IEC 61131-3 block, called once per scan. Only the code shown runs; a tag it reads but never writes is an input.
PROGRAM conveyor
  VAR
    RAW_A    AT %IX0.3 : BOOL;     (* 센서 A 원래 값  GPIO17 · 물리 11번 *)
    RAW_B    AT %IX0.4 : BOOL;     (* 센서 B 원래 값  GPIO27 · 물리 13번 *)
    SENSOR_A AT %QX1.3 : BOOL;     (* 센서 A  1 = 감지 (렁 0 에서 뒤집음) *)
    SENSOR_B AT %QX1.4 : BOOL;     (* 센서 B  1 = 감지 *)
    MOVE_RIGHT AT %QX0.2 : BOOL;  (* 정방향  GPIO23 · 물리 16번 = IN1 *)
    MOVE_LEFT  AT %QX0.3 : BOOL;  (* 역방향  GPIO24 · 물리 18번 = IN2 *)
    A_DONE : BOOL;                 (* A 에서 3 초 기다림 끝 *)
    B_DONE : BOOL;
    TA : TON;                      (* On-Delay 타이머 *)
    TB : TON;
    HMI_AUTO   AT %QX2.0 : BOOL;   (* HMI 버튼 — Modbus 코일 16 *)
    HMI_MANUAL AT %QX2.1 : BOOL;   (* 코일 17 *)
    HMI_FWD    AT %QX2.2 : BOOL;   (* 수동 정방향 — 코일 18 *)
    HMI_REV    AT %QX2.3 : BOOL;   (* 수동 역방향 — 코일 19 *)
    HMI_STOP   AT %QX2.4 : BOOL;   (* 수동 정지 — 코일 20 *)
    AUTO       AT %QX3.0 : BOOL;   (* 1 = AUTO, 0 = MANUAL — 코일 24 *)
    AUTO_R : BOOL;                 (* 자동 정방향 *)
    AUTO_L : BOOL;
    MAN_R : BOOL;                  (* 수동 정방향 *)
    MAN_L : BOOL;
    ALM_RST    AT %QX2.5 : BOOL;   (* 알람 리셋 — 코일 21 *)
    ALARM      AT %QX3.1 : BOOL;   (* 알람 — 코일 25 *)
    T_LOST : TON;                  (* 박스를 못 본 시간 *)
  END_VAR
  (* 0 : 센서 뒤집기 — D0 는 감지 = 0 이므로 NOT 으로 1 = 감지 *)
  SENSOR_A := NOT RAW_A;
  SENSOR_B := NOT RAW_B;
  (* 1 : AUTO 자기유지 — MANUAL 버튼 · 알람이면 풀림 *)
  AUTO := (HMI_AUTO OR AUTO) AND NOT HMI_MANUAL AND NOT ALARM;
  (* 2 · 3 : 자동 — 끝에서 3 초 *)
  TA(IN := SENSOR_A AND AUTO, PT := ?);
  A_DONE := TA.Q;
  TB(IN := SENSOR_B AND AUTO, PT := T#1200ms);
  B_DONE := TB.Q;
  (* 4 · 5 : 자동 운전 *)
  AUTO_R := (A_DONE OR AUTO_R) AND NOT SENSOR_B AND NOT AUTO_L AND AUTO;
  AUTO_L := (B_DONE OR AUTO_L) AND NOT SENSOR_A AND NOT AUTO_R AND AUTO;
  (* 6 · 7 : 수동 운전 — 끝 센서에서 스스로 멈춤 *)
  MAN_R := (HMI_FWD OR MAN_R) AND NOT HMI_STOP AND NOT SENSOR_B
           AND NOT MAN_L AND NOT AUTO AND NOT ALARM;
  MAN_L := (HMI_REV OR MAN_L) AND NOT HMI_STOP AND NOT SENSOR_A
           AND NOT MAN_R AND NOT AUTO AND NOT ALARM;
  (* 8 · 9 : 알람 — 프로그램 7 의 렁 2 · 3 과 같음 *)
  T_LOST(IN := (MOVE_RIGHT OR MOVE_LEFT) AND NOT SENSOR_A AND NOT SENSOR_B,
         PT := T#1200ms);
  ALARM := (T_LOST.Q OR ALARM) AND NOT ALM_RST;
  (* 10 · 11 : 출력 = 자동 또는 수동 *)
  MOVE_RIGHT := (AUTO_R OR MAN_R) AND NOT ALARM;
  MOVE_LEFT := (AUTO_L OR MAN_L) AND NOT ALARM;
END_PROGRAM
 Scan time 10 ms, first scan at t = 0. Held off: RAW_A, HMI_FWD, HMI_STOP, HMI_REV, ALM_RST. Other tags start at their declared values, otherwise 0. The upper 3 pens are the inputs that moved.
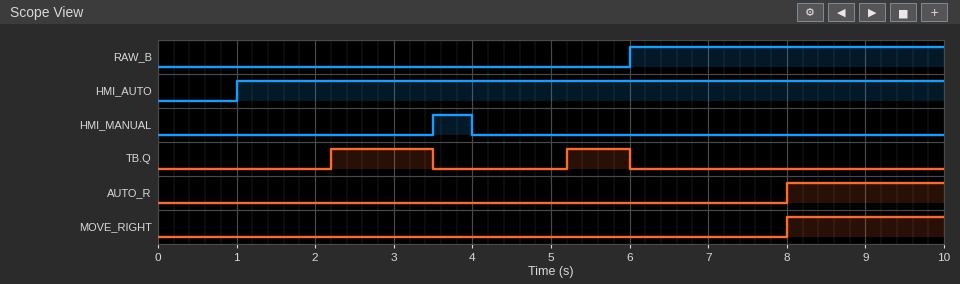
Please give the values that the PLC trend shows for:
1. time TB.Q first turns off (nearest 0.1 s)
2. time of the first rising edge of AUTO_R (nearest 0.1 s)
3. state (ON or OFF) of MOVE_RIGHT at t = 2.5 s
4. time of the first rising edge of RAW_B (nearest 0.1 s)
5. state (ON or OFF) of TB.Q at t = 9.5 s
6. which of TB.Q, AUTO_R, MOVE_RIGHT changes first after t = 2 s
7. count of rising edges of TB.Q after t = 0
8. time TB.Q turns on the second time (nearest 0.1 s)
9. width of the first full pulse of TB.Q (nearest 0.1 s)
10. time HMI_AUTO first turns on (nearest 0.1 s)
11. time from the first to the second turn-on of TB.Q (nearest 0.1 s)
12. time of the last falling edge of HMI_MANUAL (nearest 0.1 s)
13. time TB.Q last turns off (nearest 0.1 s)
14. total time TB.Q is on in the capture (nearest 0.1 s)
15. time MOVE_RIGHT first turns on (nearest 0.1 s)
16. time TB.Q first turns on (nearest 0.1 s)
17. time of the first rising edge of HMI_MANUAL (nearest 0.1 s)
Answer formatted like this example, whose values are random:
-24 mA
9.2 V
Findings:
3.5 s
8.0 s
OFF
6.0 s
OFF
TB.Q
2
5.2 s
1.3 s
1.0 s
3.0 s
4.0 s
6.0 s
2.1 s
8.0 s
2.2 s
3.5 s
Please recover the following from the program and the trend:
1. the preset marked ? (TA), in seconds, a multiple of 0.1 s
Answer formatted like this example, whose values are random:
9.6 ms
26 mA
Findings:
4.0 s
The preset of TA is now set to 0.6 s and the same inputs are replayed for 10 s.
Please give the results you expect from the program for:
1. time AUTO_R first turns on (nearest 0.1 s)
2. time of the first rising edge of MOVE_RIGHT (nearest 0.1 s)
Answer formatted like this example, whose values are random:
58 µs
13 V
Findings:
6.0 s
6.0 s
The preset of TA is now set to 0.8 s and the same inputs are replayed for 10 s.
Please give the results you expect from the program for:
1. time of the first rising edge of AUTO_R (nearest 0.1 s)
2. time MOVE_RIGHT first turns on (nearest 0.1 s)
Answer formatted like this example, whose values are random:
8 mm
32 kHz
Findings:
6.0 s
6.0 s
